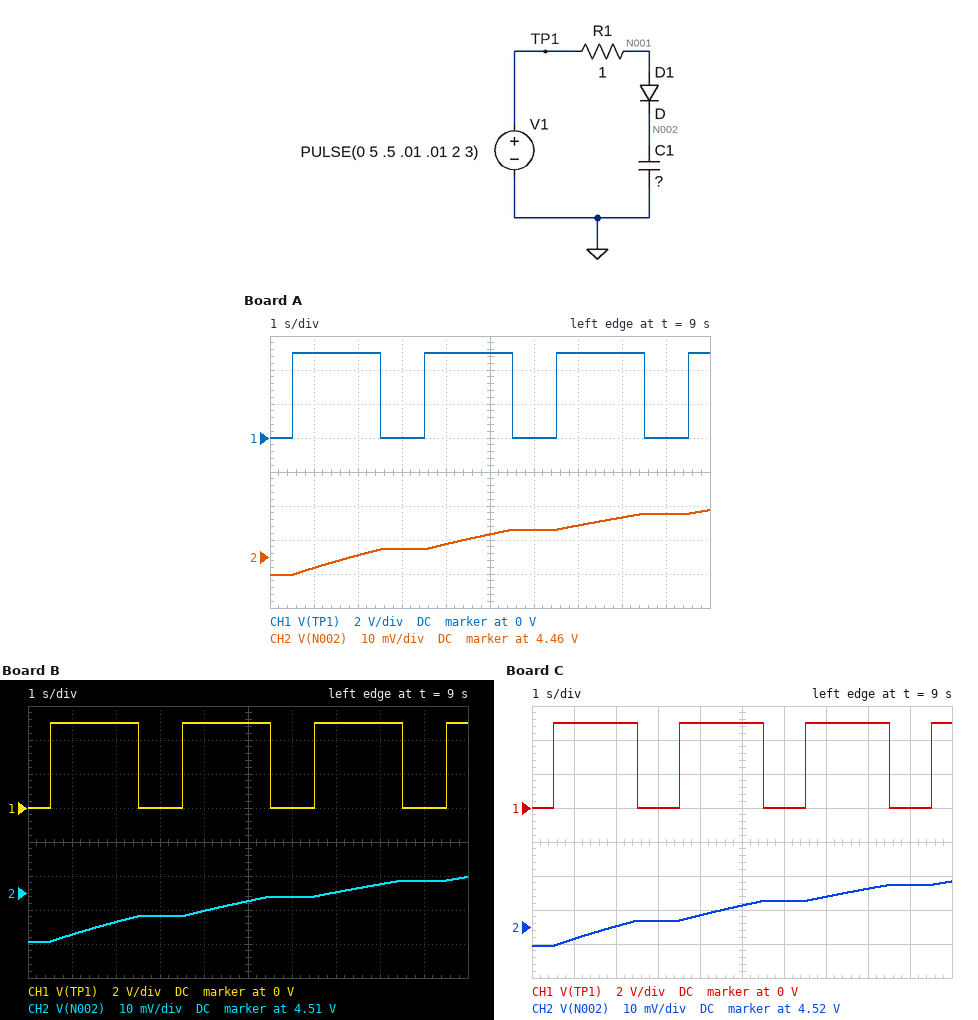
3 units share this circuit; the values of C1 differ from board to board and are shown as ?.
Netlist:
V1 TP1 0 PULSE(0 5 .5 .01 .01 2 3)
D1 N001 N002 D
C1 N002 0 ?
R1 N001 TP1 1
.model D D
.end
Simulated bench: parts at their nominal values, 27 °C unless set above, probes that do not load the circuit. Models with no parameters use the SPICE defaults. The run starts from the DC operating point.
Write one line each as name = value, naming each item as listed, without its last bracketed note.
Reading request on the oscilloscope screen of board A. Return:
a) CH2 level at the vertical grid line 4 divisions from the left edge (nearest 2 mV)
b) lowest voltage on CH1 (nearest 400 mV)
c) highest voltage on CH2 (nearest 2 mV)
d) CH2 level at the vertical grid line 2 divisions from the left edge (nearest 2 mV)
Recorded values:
CH2 level at the vertical grid line 4 divisions from the left edge = 4.464 V
lowest voltage on CH1 = 0 V
highest voltage on CH2 = 4.474 V
CH2 level at the vertical grid line 2 divisions from the left edge = 4.460 V
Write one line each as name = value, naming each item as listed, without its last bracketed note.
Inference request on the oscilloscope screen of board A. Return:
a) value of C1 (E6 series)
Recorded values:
value of C1 = 3.3 mF
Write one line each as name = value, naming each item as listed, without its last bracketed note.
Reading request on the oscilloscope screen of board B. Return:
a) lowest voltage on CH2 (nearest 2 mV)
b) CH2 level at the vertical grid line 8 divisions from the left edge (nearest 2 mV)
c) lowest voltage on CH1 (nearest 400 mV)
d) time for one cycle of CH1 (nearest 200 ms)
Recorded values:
lowest voltage on CH2 = 4.496 V
CH2 level at the vertical grid line 8 divisions from the left edge = 4.512 V
lowest voltage on CH1 = 0 V
time for one cycle of CH1 = 3.0 s
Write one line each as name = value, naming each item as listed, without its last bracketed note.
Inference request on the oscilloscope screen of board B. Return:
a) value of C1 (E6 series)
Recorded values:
value of C1 = 680 µF
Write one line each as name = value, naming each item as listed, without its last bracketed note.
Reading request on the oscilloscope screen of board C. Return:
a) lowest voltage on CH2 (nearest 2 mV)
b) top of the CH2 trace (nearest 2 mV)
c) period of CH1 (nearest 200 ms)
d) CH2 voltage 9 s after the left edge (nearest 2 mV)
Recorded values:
lowest voltage on CH2 = 4.514 V
top of the CH2 trace = 4.534 V
period of CH1 = 3.0 s
CH2 voltage 9 s after the left edge = 4.532 V
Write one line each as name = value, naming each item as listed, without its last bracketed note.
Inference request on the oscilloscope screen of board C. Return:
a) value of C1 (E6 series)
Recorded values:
value of C1 = 330 µF
